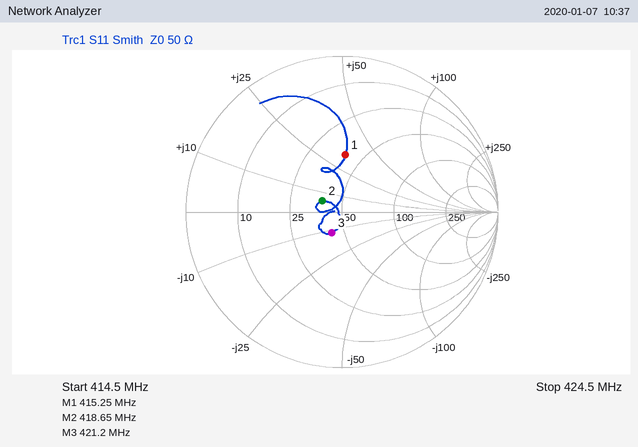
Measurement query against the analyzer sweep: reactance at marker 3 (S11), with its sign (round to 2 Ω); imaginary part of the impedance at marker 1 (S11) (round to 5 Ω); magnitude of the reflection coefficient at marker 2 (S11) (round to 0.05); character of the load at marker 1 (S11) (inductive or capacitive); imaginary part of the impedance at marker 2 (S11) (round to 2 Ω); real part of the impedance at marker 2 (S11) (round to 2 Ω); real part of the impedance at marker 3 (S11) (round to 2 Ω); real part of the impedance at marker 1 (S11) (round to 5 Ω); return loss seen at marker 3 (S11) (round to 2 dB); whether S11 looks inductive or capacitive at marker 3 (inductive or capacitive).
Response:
-12 Ω
+35 Ω
0.15
inductive
+6 Ω
38 Ω
42 Ω
40 Ω
16 dB
capacitive
